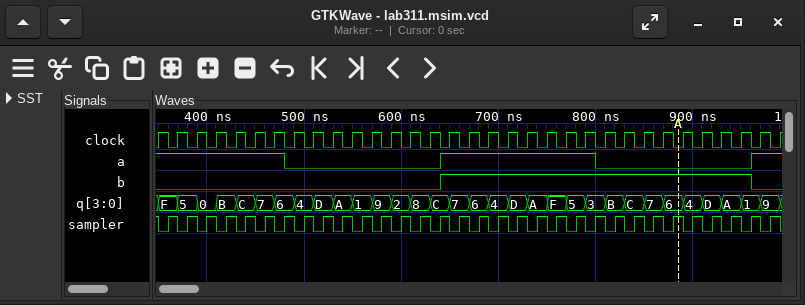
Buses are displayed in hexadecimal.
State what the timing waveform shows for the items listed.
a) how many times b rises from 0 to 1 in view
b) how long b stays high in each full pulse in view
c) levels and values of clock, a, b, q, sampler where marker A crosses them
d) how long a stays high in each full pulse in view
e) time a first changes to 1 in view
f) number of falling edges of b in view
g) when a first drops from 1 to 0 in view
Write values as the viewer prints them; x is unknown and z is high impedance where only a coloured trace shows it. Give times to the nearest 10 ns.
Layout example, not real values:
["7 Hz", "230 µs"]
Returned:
["1", "320 ns", "clock=0, a=0, b=1, q=6, sampler=1", "160 ns", "640 ns", "1", "480 ns"]
